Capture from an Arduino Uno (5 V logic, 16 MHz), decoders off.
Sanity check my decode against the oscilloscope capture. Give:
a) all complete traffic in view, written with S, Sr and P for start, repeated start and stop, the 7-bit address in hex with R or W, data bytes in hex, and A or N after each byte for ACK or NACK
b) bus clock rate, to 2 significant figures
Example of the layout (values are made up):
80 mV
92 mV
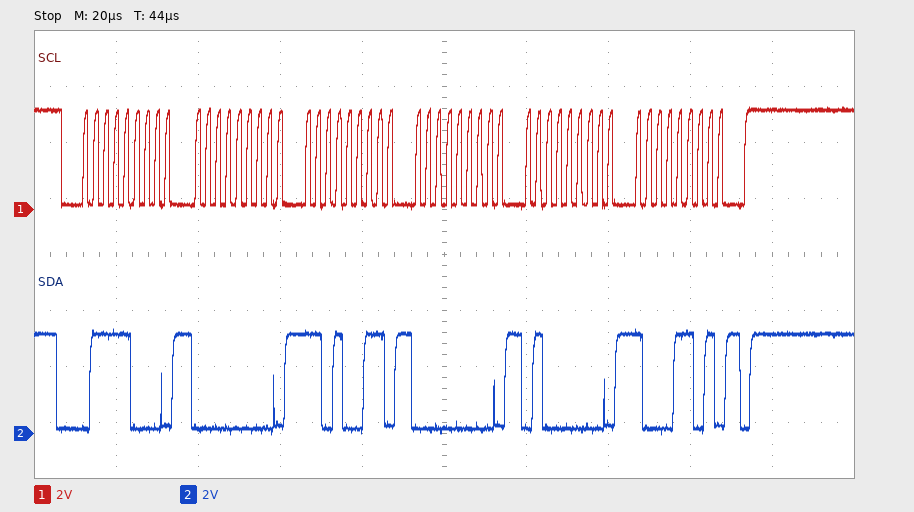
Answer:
S 3CW A 00 A D3 A 00 A 40 A 8D A P
400 kHz
